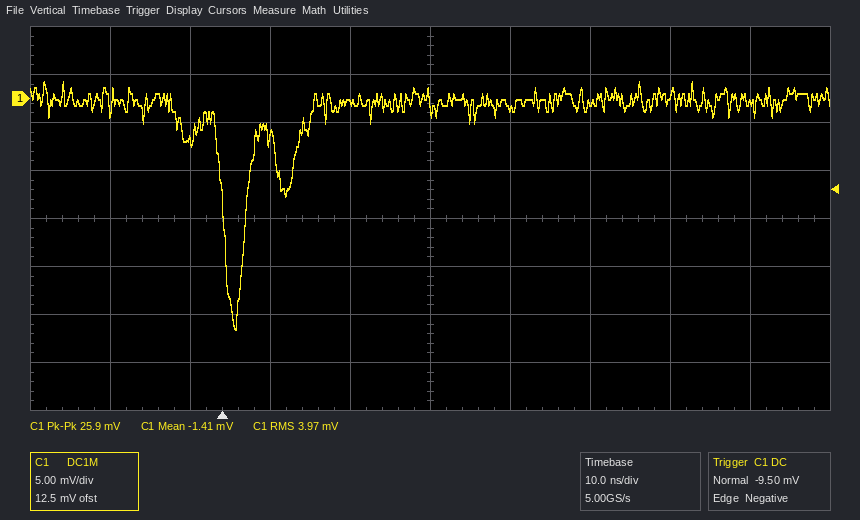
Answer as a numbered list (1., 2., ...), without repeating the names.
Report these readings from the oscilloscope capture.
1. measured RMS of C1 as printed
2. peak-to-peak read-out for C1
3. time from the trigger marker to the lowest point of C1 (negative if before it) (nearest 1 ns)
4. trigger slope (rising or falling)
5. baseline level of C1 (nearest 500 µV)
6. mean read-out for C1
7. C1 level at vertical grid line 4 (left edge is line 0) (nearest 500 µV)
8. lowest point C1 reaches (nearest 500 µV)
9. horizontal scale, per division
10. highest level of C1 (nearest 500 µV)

1. 3.97 mV
2. 25.9 mV
3. +2 ns
4. falling
5. -500 µV
6. -1.41 mV
7. -500 µV
8. -24.0 mV
9. 10 ns
10. 2.0 mV
